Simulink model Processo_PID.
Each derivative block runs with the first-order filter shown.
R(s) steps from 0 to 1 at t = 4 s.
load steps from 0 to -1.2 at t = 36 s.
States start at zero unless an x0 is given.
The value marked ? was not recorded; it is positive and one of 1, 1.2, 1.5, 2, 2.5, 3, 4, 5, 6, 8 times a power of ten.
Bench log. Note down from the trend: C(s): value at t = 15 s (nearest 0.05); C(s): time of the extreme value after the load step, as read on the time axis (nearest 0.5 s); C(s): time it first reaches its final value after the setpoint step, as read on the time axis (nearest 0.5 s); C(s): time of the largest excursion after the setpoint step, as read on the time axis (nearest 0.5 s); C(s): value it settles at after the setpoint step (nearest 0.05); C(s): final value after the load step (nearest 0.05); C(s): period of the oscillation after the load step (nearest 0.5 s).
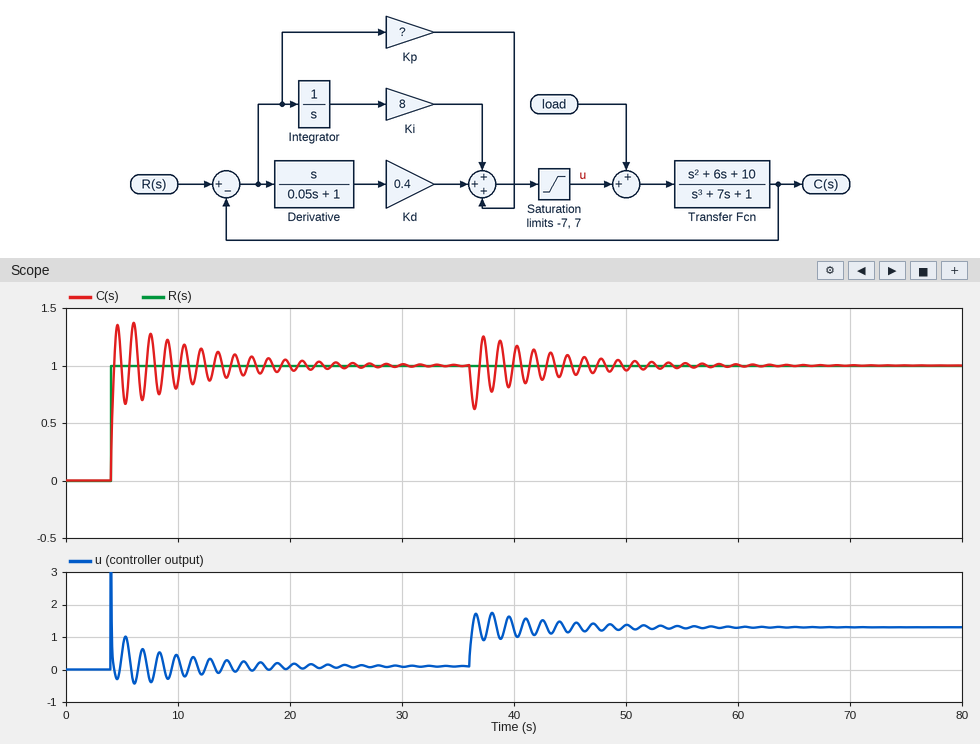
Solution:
1.10
36.5 s
4.5 s
6.0 s
1.00
1.00
1.5 s
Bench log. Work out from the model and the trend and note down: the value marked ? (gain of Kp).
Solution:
1.5
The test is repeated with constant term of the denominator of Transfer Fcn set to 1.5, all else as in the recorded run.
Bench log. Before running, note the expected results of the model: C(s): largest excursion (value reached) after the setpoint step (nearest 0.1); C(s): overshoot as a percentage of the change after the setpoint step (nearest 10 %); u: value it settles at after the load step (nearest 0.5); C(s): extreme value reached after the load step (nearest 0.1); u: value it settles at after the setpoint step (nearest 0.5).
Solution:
1.4
40 %
1.5
0.6
0.0
